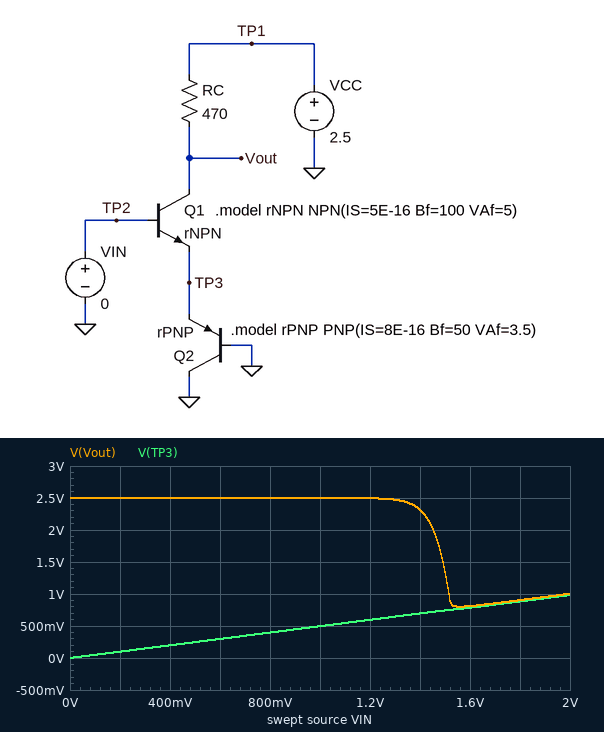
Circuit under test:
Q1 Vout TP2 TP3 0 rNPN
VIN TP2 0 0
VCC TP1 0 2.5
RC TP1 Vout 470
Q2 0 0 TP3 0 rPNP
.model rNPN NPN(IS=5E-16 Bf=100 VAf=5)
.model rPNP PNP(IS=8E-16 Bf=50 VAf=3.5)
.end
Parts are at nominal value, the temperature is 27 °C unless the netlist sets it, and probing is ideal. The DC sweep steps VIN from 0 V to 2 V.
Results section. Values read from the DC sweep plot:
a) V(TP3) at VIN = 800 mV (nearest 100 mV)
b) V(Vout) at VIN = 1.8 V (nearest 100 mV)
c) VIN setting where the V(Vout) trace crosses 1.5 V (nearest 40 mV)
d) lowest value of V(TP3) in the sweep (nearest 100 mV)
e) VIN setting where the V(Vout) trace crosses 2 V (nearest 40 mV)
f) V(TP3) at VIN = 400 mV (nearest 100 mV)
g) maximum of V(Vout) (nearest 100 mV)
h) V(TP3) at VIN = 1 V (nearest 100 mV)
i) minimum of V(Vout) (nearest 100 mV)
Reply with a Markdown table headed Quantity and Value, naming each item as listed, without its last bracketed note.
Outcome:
| Quantity | Value |
|---|---|
| V(TP3) at VIN = 800 mV | 400 mV |
| V(Vout) at VIN = 1.8 V | 900 mV |
| VIN setting where the V(Vout) trace crosses 1.5 V | 1.48 V |
| lowest value of V(TP3) in the sweep | 0 V |
| VIN setting where the V(Vout) trace crosses 2 V | 1.44 V |
| V(TP3) at VIN = 400 mV | 200 mV |
| maximum of V(Vout) | 2.5 V |
| V(TP3) at VIN = 1 V | 500 mV |
| minimum of V(Vout) | 800 mV |
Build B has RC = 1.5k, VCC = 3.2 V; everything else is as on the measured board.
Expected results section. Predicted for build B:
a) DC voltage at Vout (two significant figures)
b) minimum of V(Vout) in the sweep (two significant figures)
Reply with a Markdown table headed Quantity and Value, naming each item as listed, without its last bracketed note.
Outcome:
| Quantity | Value |
|---|---|
| DC voltage at Vout | 3.2 V |
| minimum of V(Vout) in the sweep | 780 mV |
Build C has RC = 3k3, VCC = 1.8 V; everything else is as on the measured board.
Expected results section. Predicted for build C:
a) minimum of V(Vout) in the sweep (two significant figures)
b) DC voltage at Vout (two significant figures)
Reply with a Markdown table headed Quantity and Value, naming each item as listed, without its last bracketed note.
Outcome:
| Quantity | Value |
|---|---|
| minimum of V(Vout) in the sweep | 740 mV |
| DC voltage at Vout | 1.8 V |
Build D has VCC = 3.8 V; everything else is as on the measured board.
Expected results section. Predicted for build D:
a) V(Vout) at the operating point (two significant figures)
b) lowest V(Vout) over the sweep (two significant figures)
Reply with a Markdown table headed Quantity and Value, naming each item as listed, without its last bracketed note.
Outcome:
| Quantity | Value |
|---|---|
| V(Vout) at the operating point | 3.8 V |
| lowest V(Vout) over the sweep | 820 mV |
